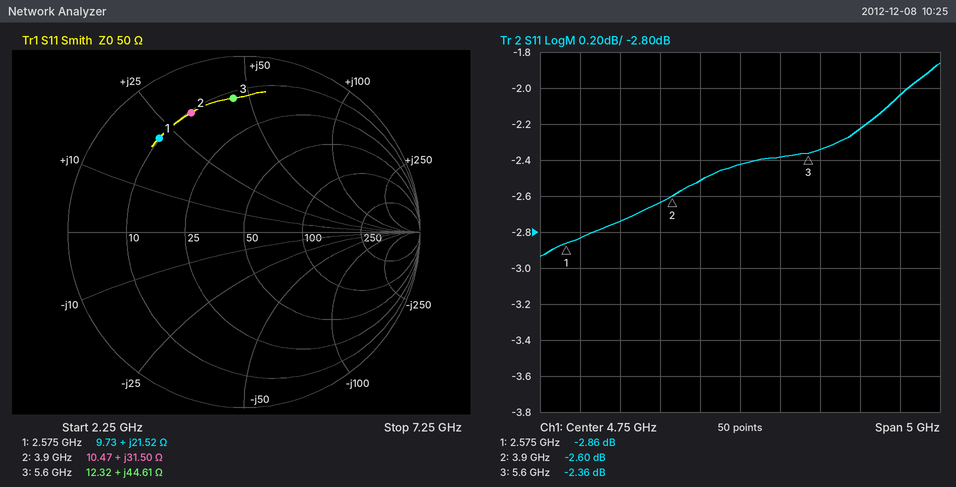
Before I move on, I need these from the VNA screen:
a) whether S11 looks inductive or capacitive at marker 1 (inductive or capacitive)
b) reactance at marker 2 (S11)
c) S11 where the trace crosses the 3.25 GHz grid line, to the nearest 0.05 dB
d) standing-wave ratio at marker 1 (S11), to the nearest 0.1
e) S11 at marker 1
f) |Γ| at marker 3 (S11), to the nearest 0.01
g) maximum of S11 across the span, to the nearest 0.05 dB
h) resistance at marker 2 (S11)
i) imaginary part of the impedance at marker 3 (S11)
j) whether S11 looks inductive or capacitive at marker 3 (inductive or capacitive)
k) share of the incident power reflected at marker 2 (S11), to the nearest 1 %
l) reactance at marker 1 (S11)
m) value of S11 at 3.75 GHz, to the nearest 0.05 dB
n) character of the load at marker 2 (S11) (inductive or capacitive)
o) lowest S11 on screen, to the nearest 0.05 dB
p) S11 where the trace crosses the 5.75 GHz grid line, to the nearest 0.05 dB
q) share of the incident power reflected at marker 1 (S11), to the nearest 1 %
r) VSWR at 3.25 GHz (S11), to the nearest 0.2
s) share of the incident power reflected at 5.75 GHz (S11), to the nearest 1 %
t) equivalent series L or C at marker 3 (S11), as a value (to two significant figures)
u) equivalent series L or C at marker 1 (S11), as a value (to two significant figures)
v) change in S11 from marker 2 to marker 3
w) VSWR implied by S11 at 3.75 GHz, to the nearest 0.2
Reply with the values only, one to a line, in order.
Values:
inductive
+31.50 Ω
-2.75 dB
6.1
-2.86 dB
0.76
-1.85 dB
10.47 Ω
+44.61 Ω
inductive
55 %
+21.52 Ω
-2.65 dB
inductive
-2.95 dB
-2.35 dB
52 %
6.4
58 %
1.3 nH
1.3 nH
0.24 dB
6.6
